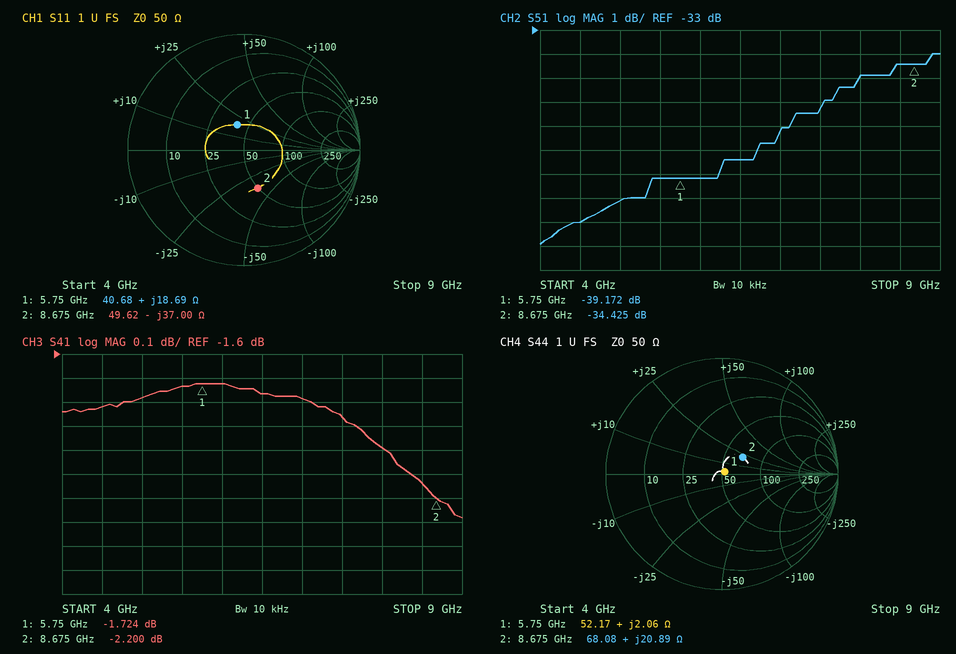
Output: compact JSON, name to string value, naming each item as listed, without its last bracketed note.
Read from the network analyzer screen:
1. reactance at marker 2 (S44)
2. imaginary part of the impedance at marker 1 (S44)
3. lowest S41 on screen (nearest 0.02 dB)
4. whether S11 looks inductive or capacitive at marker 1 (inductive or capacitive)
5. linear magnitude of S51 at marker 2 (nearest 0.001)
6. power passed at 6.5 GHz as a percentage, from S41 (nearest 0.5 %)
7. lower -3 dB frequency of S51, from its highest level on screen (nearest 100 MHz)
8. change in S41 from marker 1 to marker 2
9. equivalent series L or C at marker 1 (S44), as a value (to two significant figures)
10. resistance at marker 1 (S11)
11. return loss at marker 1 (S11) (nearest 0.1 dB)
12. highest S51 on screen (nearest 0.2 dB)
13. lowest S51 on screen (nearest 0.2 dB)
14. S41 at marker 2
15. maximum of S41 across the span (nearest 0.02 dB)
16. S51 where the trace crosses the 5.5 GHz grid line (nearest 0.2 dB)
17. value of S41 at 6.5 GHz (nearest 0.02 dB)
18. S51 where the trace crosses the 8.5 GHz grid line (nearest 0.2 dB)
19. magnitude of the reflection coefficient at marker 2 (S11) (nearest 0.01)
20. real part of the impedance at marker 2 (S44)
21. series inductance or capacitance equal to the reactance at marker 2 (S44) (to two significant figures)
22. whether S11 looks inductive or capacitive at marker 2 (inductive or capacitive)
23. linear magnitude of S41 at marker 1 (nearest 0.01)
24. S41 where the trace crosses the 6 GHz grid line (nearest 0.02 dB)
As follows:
{"reactance at marker 2": "+20.89 Ω", "imaginary part of the impedance at marker 1": "+2.06 Ω", "lowest S41 on screen": "-2.28 dB", "whether S11 looks inductive or capacitive at marker 1": "inductive", "linear magnitude of S51 at marker 2": "0.019", "power passed at 6.5 GHz as a percentage, from S41": "66.5 %", "lower -3 dB frequency of S51, from its highest level on screen": "7.1 GHz", "change in S41 from marker 1 to marker 2": "-0.476 dB", "equivalent series L or C at marker 1 (S44), as a value": "57 pH", "resistance at marker 1": "40.68 Ω", "return loss at marker 1 (S11)": "12.9 dB", "highest S51 on screen": "-34.0 dB", "lowest S51 on screen": "-42.0 dB", "S41 at marker 2": "-2.200 dB", "maximum of S41 across the span": "-1.72 dB", "S51 where the trace crosses the 5.5 GHz grid line": "-39.2 dB", "value of S41 at 6.5 GHz": "-1.76 dB", "S51 where the trace crosses the 8.5 GHz grid line": "-34.4 dB", "magnitude of the reflection coefficient at marker 2 (S11)": "0.35", "real part of the impedance at marker 2": "68.08 Ω", "series inductance or capacitance equal to the reactance at marker 2 (S44)": "380 pH", "whether S11 looks inductive or capacitive at marker 2": "capacitive", "linear magnitude of S41 at marker 1": "0.82", "S41 where the trace crosses the 6 GHz grid line": "-1.72 dB"}
